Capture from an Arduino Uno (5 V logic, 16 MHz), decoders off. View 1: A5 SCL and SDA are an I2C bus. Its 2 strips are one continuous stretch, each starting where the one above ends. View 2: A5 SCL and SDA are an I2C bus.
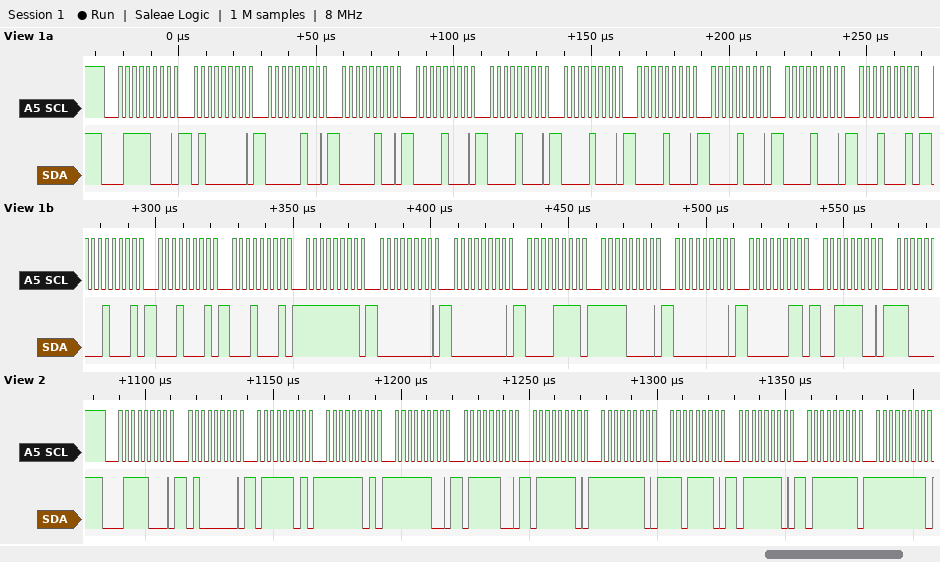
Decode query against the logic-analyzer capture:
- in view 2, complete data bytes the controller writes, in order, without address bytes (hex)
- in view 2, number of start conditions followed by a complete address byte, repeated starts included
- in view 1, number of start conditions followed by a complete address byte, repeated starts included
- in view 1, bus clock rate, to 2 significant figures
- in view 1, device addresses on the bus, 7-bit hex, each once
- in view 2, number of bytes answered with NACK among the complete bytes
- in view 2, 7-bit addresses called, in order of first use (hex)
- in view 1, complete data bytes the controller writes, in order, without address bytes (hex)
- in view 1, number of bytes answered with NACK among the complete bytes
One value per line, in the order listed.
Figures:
40 7D FD FC 7C 7E FE DE 7E 7F FF
1
1
400 kHz
0x3C
0
0x3C
40 04 04 08 08 08 08 08 08 11 11 11 11 FF 00 00 0F F0 00 03 3C
0
